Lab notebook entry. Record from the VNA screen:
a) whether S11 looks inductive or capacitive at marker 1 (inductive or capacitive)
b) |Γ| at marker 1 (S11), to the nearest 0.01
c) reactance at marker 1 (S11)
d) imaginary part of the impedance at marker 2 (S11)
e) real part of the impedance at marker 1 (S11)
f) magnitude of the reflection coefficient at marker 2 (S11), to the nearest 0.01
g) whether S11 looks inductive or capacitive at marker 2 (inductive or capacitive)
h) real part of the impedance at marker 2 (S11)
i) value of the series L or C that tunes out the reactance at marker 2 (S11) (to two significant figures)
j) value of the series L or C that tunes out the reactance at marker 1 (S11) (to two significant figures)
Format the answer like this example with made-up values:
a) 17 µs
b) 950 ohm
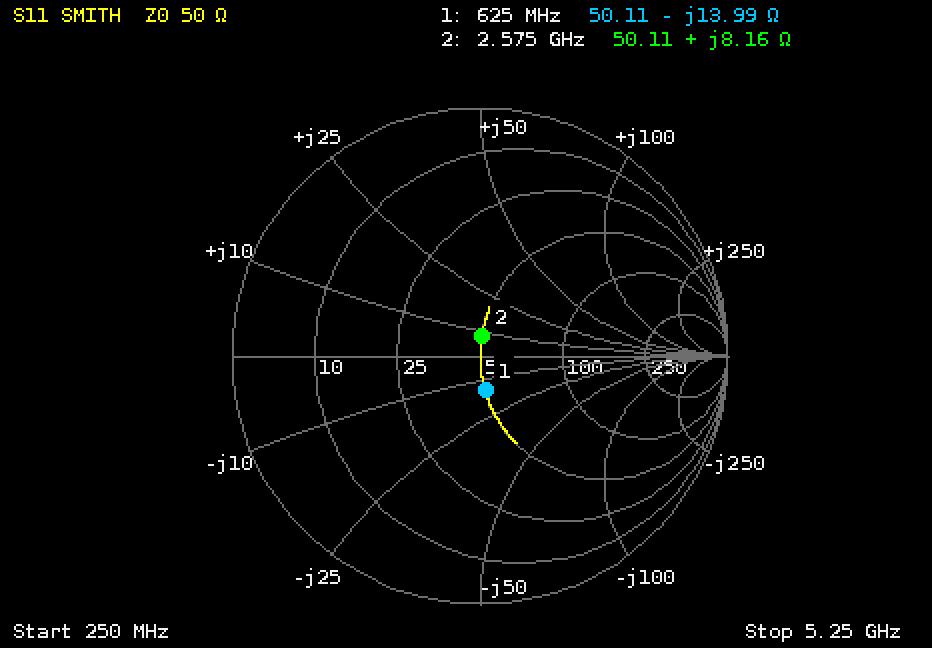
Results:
a) capacitive
b) 0.14
c) -13.99 Ω
d) +8.16 Ω
e) 50.11 Ω
f) 0.08
g) inductive
h) 50.11 Ω
i) 7.6 pF
j) 3.6 nH
